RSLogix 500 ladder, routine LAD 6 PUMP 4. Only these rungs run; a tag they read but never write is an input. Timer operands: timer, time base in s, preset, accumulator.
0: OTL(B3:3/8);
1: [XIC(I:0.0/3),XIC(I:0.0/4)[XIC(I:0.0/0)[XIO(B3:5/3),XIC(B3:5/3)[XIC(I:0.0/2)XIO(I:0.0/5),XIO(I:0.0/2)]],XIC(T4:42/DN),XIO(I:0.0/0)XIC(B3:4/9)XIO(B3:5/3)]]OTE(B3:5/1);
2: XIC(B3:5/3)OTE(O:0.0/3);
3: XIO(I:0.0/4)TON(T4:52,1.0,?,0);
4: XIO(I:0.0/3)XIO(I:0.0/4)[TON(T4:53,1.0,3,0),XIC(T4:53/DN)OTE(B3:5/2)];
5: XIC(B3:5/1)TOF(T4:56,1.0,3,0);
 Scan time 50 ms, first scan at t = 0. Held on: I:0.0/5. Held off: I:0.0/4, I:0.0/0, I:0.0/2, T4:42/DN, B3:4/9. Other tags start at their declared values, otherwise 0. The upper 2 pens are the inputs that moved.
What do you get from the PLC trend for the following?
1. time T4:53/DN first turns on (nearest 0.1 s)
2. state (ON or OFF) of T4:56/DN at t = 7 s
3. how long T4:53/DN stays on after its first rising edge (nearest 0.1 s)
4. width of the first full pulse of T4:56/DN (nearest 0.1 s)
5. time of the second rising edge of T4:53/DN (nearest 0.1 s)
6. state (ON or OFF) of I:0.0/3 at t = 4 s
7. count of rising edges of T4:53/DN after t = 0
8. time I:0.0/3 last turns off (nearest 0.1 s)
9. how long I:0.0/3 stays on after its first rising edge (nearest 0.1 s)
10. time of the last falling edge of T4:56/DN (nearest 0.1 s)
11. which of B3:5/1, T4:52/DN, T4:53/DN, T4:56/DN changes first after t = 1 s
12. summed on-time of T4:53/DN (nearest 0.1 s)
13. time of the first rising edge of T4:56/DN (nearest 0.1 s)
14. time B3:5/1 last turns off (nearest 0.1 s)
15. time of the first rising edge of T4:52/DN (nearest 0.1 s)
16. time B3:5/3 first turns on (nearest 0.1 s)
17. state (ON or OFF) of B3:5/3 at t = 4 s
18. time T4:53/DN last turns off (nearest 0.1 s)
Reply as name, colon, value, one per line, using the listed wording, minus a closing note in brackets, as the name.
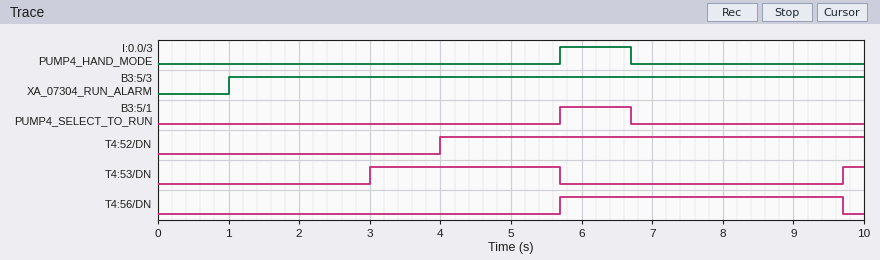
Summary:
time T4:53/DN first turns on: 3.0 s
state (ON or OFF) of T4:56/DN at t = 7 s: ON
how long T4:53/DN stays on after its first rising edge: 2.7 s
width of the first full pulse of T4:56/DN: 4.0 s
time of the second rising edge of T4:53/DN: 9.7 s
state (ON or OFF) of I:0.0/3 at t = 4 s: OFF
count of rising edges of T4:53/DN after t = 0: 2
time I:0.0/3 last turns off: 6.7 s
how long I:0.0/3 stays on after its first rising edge: 1.0 s
time of the last falling edge of T4:56/DN: 9.7 s
which of B3:5/1, T4:52/DN, T4:53/DN, T4:56/DN changes first after t = 1 s: T4:53/DN
summed on-time of T4:53/DN: 3.0 s
time of the first rising edge of T4:56/DN: 5.7 s
time B3:5/1 last turns off: 6.7 s
time of the first rising edge of T4:52/DN: 4.0 s
time B3:5/3 first turns on: 1.0 s
state (ON or OFF) of B3:5/3 at t = 4 s: ON
time T4:53/DN last turns off: 5.7 s
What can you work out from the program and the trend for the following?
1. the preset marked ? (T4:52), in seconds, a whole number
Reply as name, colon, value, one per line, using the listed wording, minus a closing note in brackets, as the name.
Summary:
the preset marked ? (T4:52), in seconds, a whole number: 4 s
